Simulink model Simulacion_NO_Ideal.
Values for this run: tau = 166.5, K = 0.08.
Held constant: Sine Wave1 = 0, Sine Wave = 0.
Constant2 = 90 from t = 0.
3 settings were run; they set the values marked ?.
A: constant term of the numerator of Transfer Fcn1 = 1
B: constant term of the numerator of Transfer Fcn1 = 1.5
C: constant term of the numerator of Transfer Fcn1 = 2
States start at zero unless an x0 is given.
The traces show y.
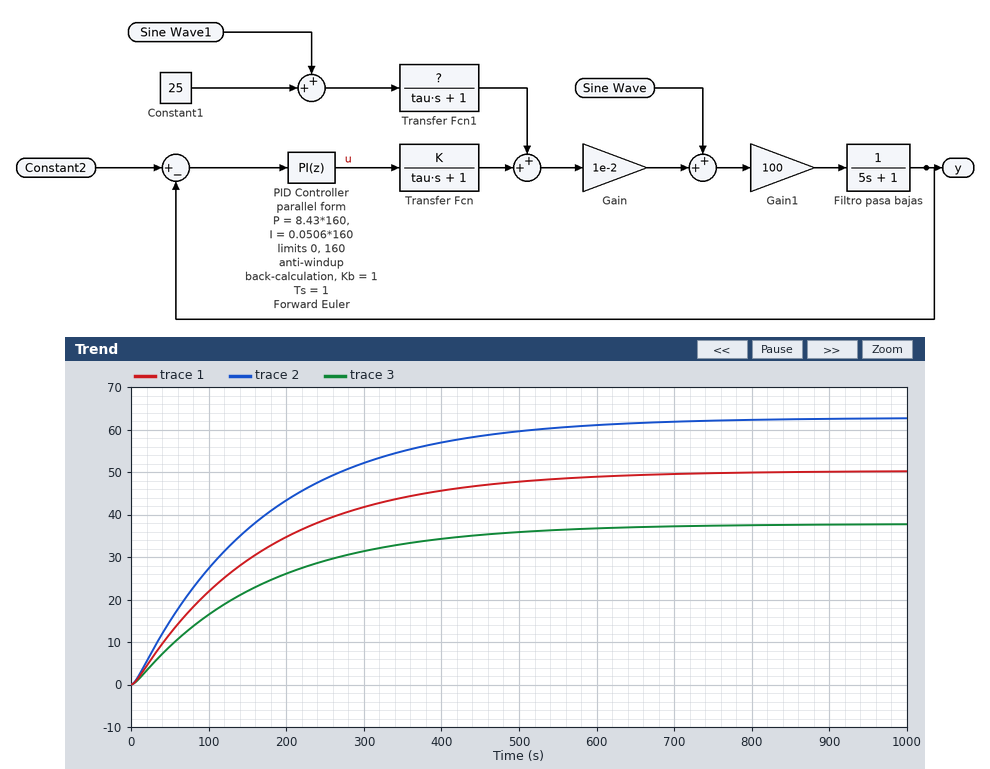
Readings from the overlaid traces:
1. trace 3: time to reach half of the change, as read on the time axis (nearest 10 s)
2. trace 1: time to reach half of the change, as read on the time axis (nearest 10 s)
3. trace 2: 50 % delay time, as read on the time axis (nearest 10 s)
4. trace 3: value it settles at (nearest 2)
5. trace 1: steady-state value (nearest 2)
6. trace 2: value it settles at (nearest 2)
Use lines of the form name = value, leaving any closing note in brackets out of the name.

trace 3: time to reach half of the change, as read on the time axis = 120 s
trace 1: time to reach half of the change, as read on the time axis = 120 s
trace 2: 50 % delay time, as read on the time axis = 120 s
trace 3: value it settles at = 38
trace 1: steady-state value = 50
trace 2: value it settles at = 62
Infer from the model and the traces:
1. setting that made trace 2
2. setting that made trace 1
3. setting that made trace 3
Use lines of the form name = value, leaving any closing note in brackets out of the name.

setting that made trace 2 = C
setting that made trace 1 = B
setting that made trace 3 = A
